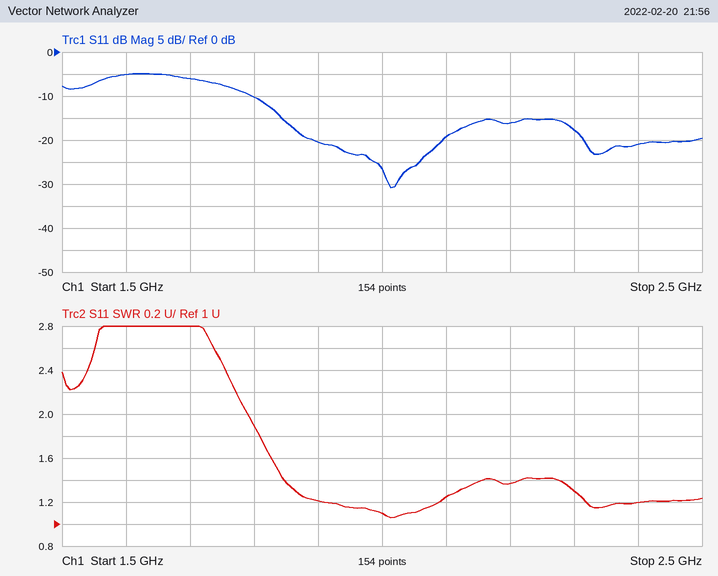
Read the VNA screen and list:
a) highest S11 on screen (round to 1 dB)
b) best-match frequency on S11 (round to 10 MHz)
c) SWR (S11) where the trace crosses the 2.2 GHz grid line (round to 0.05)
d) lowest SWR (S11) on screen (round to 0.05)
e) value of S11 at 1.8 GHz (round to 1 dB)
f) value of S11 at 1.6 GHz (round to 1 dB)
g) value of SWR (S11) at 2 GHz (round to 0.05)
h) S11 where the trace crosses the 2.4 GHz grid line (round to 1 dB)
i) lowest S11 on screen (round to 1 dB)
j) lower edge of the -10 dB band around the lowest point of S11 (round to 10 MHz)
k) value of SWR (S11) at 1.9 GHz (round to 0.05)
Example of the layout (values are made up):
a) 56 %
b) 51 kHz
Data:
a) -5 dB
b) 2.01 GHz
c) 1.35
d) 1.05
e) -10 dB
f) -5 dB
g) 1.10
h) -21 dB
i) -31 dB
j) 1.80 GHz
k) 1.20
